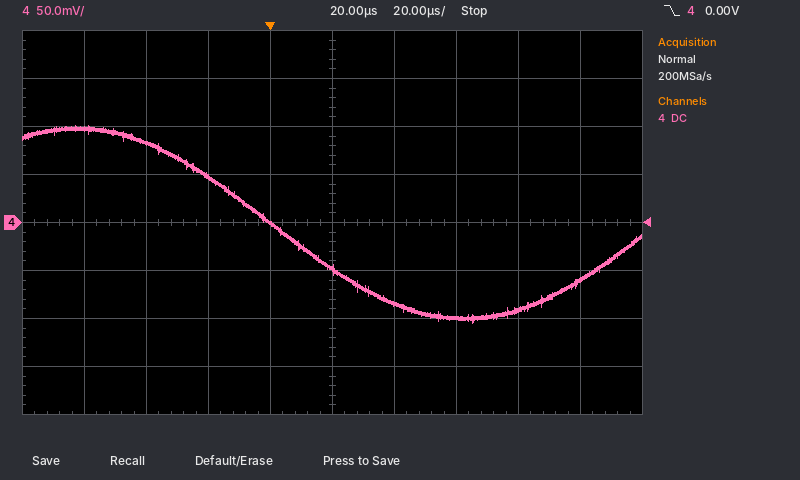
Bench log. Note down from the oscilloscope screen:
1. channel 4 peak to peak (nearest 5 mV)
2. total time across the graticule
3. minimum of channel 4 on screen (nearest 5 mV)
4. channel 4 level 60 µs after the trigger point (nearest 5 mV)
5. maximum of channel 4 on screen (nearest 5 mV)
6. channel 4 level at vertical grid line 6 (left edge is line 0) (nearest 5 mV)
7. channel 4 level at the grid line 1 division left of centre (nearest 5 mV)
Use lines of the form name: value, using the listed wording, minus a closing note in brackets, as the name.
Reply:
channel 4 peak to peak: 205 mV
total time across the graticule: 200 µs
minimum of channel 4 on screen: -105 mV
channel 4 level 60 µs after the trigger point: -100 mV
maximum of channel 4 on screen: 100 mV
channel 4 level at vertical grid line 6 (left edge is line 0): -85 mV
channel 4 level at the grid line 1 division left of centre: 0 mV
